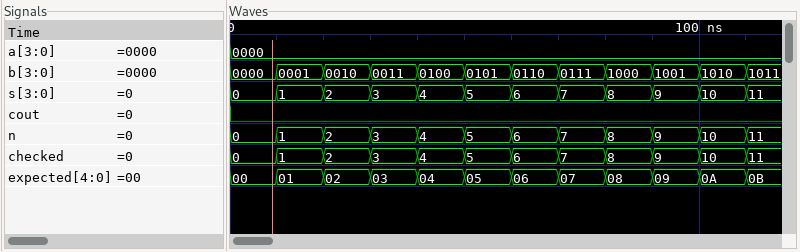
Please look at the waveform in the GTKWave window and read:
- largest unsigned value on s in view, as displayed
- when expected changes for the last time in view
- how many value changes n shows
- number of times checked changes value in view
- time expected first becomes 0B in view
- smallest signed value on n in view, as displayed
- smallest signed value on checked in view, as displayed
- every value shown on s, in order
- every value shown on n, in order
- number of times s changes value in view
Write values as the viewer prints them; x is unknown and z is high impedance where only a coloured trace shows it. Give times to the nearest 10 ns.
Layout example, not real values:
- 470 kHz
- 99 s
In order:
- 11
- 110 ns
- 11
- 11
- 110 ns
- 0
- 0
- 0, 1, 2, 3, 4, 5, 6, 7, 8, 9, 10, 11
- 0, 1, 2, 3, 4, 5, 6, 7, 8, 9, 10, 11
- 11
